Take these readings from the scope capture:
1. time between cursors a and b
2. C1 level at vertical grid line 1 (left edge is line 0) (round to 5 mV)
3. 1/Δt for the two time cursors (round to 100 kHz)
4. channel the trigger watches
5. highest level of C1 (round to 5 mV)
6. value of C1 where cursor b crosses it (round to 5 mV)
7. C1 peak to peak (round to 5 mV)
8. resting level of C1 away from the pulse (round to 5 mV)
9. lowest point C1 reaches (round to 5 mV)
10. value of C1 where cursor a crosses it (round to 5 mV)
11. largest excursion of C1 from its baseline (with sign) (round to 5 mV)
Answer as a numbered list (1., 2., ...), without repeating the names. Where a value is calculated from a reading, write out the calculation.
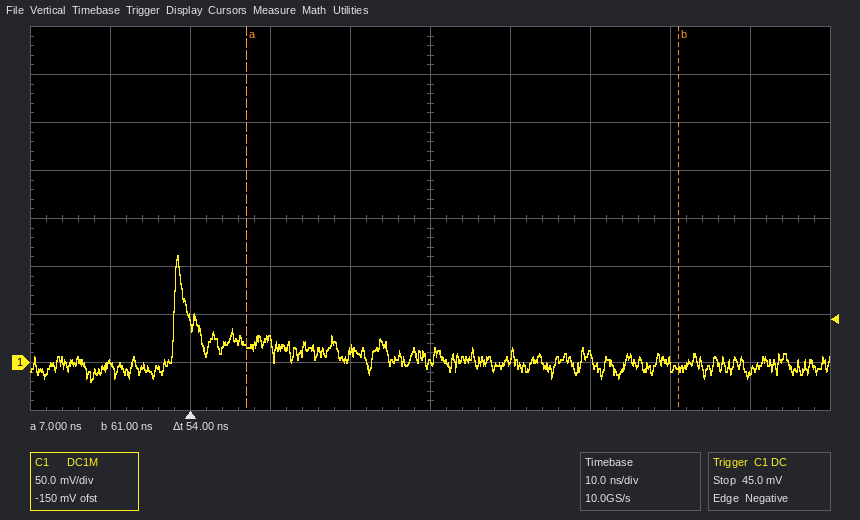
1. 54 ns
2. 0 mV
3. 1 / 54 ns ≈ 18.5 MHz
4. C1
5. 110 mV
6. -5 mV
7. 110 mV − (-20 mV) = 130 mV
8. 0 mV
9. -20 mV
10. 20 mV
11. 110 mV − (0 mV) = +110 mV
